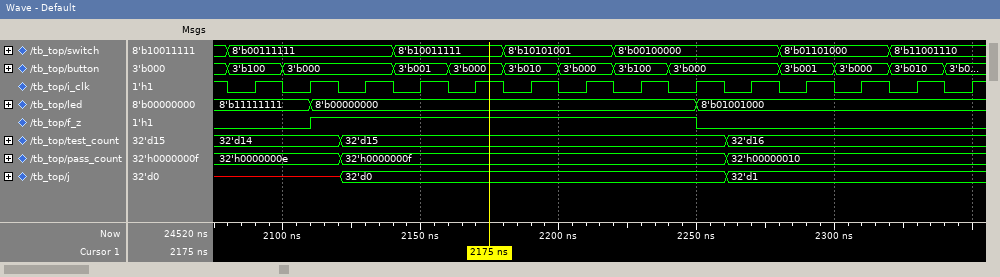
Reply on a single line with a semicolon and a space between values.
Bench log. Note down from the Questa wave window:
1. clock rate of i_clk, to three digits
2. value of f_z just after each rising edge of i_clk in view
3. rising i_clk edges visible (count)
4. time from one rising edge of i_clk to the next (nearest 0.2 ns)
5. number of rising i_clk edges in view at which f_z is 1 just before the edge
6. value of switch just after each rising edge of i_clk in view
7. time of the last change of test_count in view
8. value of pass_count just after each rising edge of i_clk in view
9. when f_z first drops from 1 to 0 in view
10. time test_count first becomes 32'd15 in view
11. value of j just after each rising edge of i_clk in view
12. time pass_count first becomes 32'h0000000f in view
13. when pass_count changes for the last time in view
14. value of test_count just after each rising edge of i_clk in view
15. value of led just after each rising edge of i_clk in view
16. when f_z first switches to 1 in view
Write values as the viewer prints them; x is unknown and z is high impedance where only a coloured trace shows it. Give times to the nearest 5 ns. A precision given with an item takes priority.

50.0 MHz; 0 1 1 1 1 1 1 1 0 0 0 0 0 0; 14; 20 ns; 7; 8'b00111111, 8'b00111111, 8'b00111111, 8'b10011111, 8'b10011111, 8'b10101001, 8'b10101001, 8'b00100000, 8'b00100000, 8'b00100000, 8'b01101000, 8'b01101000, 8'b11001110, 8'b11001110; 2260 ns; 32'h0000000e, 32'h0000000e, 32'h0000000f, 32'h0000000f, 32'h0000000f, 32'h0000000f, 32'h0000000f, 32'h0000000f, 32'h0000000f, 32'h00000010, 32'h00000010, 32'h00000010, 32'h00000010, 32'h00000010; 2250 ns; 2120 ns; x, x, 32'd0, 32'd0, 32'd0, 32'd0, 32'd0, 32'd0, 32'd0, 32'd1, 32'd1, 32'd1, 32'd1, 32'd1; 2120 ns; 2260 ns; 32'd14, 32'd14, 32'd15, 32'd15, 32'd15, 32'd15, 32'd15, 32'd15, 32'd15, 32'd16, 32'd16, 32'd16, 32'd16, 32'd16; 8'b11111111, 8'b00000000, 8'b00000000, 8'b00000000, 8'b00000000, 8'b00000000, 8'b00000000, 8'b00000000, 8'b01001000, 8'b01001000, 8'b01001000, 8'b01001000, 8'b01001000, 8'b01001000; 2110 ns
